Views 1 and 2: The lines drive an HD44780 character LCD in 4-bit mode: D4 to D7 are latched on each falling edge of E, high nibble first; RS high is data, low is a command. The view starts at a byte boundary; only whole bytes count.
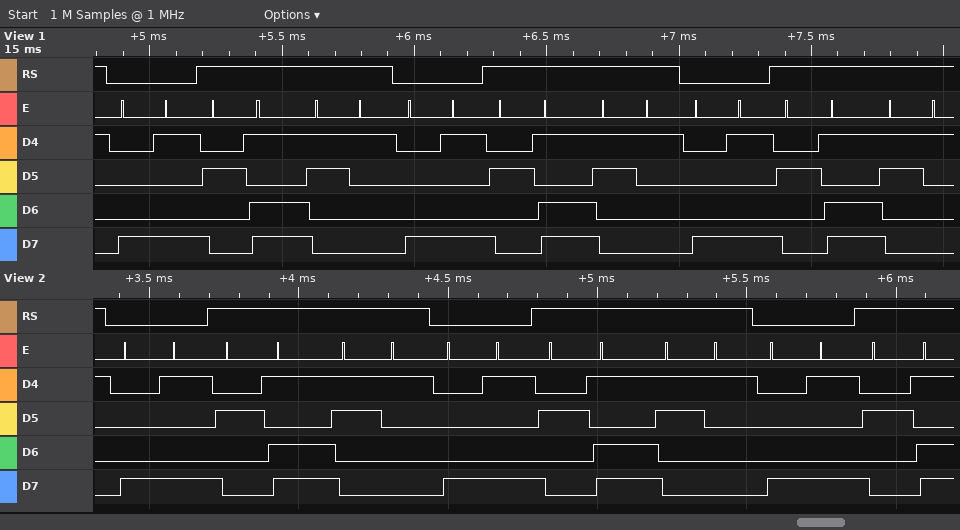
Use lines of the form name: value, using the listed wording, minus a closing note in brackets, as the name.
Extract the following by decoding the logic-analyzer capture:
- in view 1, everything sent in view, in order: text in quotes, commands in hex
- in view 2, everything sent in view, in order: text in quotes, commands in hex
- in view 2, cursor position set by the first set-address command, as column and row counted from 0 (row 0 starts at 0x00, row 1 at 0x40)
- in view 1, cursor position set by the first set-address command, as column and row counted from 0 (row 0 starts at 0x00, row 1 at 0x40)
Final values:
in view 1, everything sent in view, in order: text in quotes, commands in hex: 0x89 "-1" 0x89 "-1" 0x89 "-1"
in view 2, everything sent in view, in order: text in quotes, commands in hex: 0x89 "-1" 0x89 "-1" 0x89 "-"
in view 2, cursor position set by the first set-address command, as column and row counted from 0: column 9, row 0
in view 1, cursor position set by the first set-address command, as column and row counted from 0: column 9, row 0
